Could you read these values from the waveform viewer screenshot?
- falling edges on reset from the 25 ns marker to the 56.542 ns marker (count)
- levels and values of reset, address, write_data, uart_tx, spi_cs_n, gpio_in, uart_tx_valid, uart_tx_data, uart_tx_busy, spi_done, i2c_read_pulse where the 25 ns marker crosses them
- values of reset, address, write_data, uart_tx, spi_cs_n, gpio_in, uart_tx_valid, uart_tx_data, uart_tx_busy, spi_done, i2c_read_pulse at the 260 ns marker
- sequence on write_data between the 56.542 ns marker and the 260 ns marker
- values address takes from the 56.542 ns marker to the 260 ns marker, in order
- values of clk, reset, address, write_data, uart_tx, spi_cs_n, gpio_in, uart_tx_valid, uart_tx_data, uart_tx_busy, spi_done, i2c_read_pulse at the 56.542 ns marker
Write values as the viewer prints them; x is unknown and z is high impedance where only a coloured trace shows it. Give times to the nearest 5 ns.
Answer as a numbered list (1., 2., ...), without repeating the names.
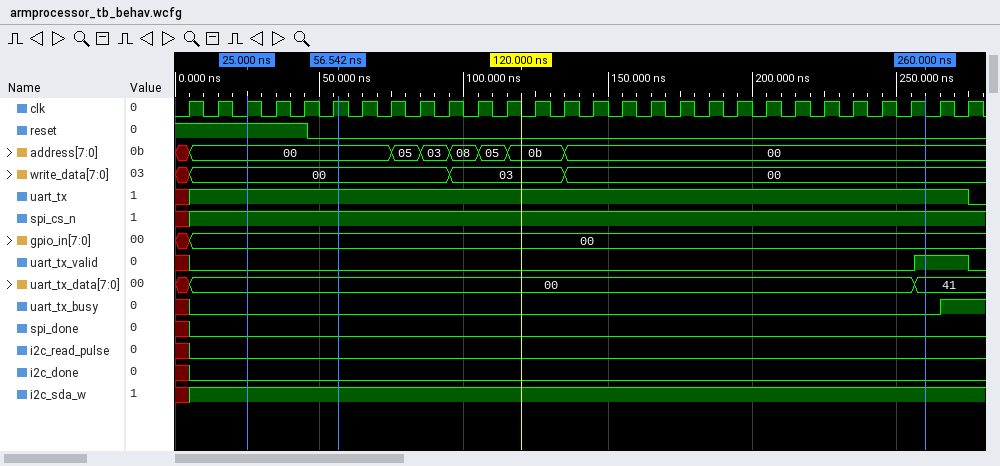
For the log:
1. 1
2. reset=1, address=00, write_data=00, uart_tx=1, spi_cs_n=1, gpio_in=00, uart_tx_valid=0, uart_tx_data=00, uart_tx_busy=0, spi_done=0, i2c_read_pulse=0
3. reset=0, address=00, write_data=00, uart_tx=1, spi_cs_n=1, gpio_in=00, uart_tx_valid=1, uart_tx_data=41, uart_tx_busy=0, spi_done=0, i2c_read_pulse=0
4. 00, 03, 00
5. 00, 05, 03, 08, 05, 0b, 00
6. clk=1, reset=0, address=00, write_data=00, uart_tx=1, spi_cs_n=1, gpio_in=00, uart_tx_valid=0, uart_tx_data=00, uart_tx_busy=0, spi_done=0, i2c_read_pulse=0
